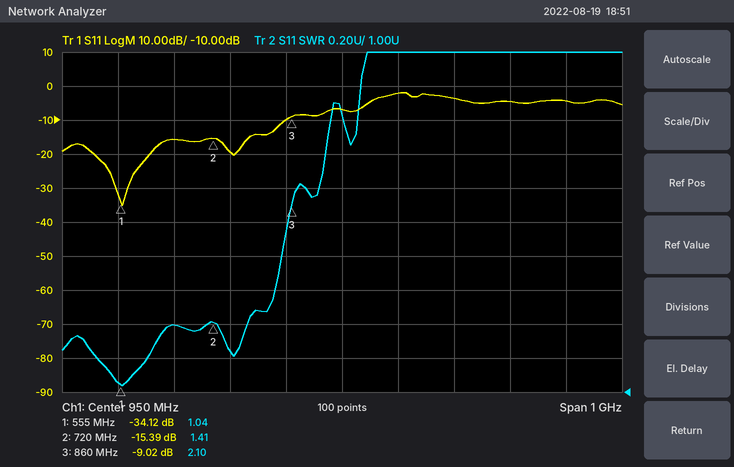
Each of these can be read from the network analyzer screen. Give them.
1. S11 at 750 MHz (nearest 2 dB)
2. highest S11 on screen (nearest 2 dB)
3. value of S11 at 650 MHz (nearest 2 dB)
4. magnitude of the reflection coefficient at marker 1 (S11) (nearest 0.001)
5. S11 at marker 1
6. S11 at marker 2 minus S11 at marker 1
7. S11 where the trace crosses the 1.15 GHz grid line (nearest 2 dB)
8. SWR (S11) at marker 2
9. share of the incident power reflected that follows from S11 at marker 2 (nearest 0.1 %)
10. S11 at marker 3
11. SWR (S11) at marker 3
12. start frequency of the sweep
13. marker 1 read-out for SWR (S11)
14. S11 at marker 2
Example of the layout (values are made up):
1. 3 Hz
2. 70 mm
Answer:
1. -20 dB
2. -2 dB
3. -16 dB
4. 0.020
5. -34.12 dB
6. 18.73 dB
7. -4 dB
8. 1.41
9. 2.9 %
10. -9.02 dB
11. 2.10
12. 450 MHz
13. 1.04
14. -15.39 dB
